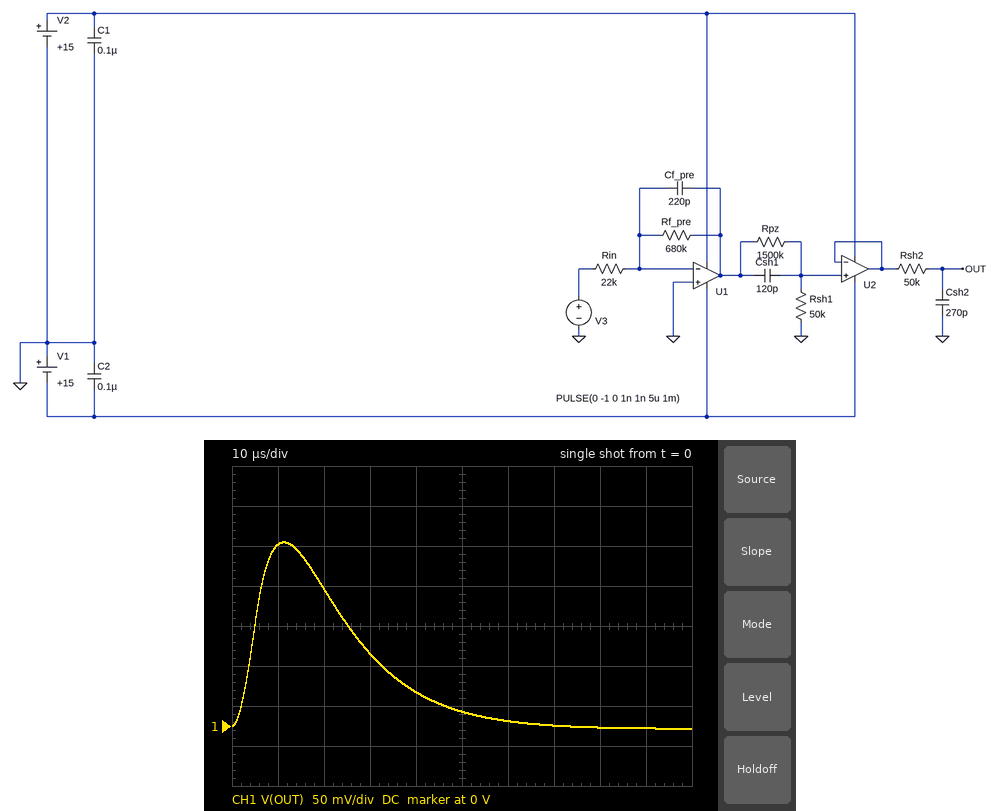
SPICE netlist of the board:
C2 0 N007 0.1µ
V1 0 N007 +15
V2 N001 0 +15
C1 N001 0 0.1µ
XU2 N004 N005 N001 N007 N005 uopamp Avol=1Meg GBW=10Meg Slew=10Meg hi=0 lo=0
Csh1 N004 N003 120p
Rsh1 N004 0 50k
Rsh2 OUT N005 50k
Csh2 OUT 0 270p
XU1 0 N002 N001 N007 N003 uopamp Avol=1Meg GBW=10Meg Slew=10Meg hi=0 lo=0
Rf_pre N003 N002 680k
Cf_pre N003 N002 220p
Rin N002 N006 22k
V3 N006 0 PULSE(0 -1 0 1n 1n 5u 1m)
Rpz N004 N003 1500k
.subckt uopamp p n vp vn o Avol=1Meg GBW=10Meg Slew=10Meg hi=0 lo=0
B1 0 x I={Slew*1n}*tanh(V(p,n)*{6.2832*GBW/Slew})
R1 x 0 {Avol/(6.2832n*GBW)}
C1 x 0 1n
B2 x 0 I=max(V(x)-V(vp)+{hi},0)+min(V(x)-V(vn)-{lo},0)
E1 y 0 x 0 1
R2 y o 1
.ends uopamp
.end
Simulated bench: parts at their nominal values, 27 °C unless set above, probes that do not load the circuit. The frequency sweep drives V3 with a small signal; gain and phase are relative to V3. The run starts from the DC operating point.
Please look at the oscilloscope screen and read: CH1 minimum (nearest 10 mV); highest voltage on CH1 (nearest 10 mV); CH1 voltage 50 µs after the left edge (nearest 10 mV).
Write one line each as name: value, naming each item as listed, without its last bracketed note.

CH1 minimum: 0 V
highest voltage on CH1: 230 mV
CH1 voltage 50 µs after the left edge: 20 mV
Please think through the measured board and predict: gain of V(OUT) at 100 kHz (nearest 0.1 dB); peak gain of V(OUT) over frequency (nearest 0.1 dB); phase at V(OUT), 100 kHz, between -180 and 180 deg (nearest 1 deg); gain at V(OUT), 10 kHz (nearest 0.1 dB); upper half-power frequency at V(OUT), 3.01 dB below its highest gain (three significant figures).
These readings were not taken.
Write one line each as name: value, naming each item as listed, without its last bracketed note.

gain of V(OUT) at 100 kHz: -28.6 dB
peak gain of V(OUT) over frequency: 1.1 dB
phase at V(OUT), 100 kHz, between -180 and 180 deg: 21 deg
gain at V(OUT), 10 kHz: -1.4 dB
upper half-power frequency at V(OUT), 3.01 dB below its highest gain: 11.1 kHz
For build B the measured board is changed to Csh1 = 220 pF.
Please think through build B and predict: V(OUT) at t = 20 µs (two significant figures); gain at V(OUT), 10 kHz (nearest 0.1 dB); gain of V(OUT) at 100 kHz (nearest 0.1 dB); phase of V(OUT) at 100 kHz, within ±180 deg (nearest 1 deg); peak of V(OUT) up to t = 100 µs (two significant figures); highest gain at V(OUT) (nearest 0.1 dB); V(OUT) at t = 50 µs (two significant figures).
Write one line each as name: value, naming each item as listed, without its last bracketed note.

V(OUT) at t = 20 µs: 290 mV
gain at V(OUT), 10 kHz: 2.8 dB
gain of V(OUT) at 100 kHz: -28.4 dB
phase of V(OUT) at 100 kHz, within ±180 deg: 14 deg
peak of V(OUT) up to t = 100 µs: 320 mV
highest gain at V(OUT): 6.0 dB
V(OUT) at t = 50 µs: 40 mV
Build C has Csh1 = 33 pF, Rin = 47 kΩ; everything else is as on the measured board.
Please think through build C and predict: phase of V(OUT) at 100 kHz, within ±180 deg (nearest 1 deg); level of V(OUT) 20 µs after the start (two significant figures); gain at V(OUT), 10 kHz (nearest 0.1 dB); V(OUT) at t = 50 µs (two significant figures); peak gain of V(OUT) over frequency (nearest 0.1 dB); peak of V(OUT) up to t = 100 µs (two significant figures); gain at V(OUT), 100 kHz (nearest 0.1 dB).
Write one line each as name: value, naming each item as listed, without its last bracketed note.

phase of V(OUT) at 100 kHz, within ±180 deg: 49 deg
level of V(OUT) 20 µs after the start: 25 mV
gain at V(OUT), 10 kHz: -18.3 dB
V(OUT) at t = 50 µs: 10 mV
peak gain of V(OUT) over frequency: -6.6 dB
peak of V(OUT) up to t = 100 µs: 43 mV
gain at V(OUT), 100 kHz: -37.9 dB
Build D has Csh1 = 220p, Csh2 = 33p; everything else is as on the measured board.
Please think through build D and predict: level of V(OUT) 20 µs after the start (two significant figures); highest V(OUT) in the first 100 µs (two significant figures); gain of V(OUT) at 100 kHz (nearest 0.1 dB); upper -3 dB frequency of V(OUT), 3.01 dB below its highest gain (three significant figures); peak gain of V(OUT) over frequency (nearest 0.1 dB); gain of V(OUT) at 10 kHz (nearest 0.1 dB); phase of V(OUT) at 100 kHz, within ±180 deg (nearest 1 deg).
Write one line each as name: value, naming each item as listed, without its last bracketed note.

level of V(OUT) 20 µs after the start: 210 mV
highest V(OUT) in the first 100 µs: 680 mV
gain of V(OUT) at 100 kHz: -13.0 dB
upper -3 dB frequency of V(OUT), 3.01 dB below its highest gain: 16.3 kHz
peak gain of V(OUT) over frequency: 6.3 dB
gain of V(OUT) at 10 kHz: 5.1 dB
phase of V(OUT) at 100 kHz, within ±180 deg: 52 deg
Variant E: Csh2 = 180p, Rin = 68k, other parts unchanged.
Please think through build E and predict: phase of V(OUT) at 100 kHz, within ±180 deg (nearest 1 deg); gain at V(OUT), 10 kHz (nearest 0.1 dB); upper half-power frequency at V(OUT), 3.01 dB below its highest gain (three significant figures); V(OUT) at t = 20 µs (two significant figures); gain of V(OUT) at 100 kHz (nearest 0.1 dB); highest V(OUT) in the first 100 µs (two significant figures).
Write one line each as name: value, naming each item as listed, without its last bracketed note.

phase of V(OUT) at 100 kHz, within ±180 deg: 24 deg
gain at V(OUT), 10 kHz: -10.0 dB
upper half-power frequency at V(OUT), 3.01 dB below its highest gain: 14.6 kHz
V(OUT) at t = 20 µs: 56 mV
gain of V(OUT) at 100 kHz: -35.0 dB
highest V(OUT) in the first 100 µs: 95 mV
